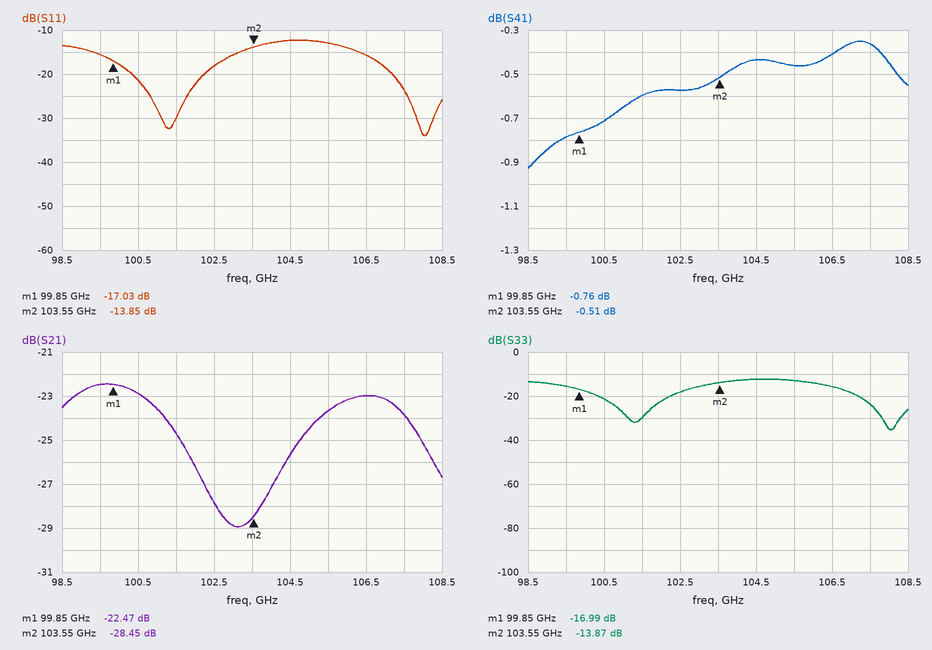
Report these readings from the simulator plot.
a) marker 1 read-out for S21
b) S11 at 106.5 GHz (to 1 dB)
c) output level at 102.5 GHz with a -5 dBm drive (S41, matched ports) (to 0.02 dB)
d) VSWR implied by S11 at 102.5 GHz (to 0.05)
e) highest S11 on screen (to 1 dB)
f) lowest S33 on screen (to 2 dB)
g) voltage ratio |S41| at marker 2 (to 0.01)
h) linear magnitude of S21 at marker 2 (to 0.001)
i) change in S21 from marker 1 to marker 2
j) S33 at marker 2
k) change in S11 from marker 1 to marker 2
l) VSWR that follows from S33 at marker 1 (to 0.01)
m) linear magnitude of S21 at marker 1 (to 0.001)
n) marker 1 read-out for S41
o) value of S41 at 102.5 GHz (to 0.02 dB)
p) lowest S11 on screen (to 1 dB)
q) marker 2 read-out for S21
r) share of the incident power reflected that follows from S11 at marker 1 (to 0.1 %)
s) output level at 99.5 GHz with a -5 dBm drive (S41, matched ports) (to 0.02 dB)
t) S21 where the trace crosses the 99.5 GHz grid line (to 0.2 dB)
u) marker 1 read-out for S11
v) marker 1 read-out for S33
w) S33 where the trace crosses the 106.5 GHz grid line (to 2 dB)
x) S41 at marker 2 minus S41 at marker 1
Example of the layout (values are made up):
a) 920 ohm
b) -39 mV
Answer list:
a) -22.47 dB
b) -16 dB
c) -5.58 dBm
d) 1.30
e) -12 dB
f) -36 dB
g) 0.94
h) 0.038
i) -5.98 dB
j) -13.87 dB
k) 3.18 dB
l) 1.33
m) 0.075
n) -0.76 dB
o) -0.58 dB
p) -34 dB
q) -28.45 dB
r) 2.0 %
s) -5.78 dBm
t) -22.4 dB
u) -17.03 dB
v) -16.99 dB
w) -16 dB
x) 0.25 dB
